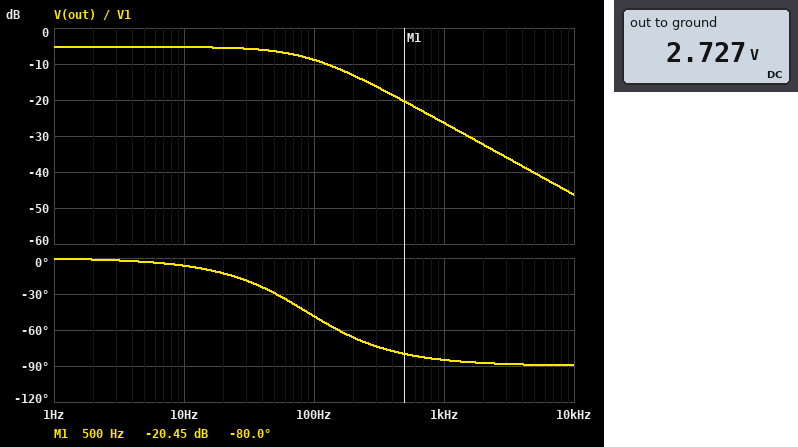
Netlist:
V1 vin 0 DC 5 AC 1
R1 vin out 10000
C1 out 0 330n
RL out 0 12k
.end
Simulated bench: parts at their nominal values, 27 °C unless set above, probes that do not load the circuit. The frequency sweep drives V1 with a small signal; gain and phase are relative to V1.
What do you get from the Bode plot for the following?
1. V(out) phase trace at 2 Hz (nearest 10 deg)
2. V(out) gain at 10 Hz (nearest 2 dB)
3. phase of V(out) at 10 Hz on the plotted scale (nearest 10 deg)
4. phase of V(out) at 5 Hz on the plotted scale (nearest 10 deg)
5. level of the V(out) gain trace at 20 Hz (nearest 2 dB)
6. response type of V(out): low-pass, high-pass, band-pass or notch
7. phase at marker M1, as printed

0 deg
-6 dB
-10 deg
0 deg
-6 dB
low-pass
-80.0 deg
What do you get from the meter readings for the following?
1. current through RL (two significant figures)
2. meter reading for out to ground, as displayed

230 µA
2.727 V
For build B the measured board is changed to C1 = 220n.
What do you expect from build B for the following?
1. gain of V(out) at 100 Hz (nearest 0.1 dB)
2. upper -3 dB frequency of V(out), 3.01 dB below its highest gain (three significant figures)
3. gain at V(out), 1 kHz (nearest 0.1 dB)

-7.2 dB
133 Hz
-22.9 dB
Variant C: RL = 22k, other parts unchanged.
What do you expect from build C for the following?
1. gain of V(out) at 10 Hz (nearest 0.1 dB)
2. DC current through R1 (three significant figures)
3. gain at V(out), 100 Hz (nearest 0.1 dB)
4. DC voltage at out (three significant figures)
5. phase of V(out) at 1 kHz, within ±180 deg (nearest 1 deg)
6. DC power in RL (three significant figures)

-3.3 dB
156 µA
-8.1 dB
3.44 V
-86 deg
537 µW
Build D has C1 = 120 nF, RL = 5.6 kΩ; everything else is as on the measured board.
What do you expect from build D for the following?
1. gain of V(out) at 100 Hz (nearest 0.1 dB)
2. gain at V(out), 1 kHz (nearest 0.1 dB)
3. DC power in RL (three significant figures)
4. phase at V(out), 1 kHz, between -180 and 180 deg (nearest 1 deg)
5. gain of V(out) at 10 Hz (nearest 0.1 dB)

-9.2 dB
-18.1 dB
575 µW
-70 deg
-8.9 dB
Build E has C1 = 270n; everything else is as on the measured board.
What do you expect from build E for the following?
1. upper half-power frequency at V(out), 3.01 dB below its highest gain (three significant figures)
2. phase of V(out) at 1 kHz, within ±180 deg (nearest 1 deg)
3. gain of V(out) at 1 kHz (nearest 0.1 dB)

108 Hz
-84 deg
-24.6 dB
